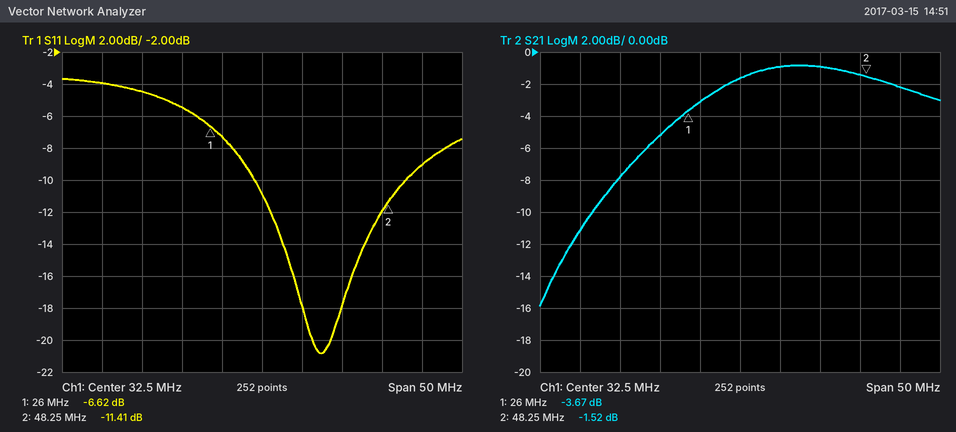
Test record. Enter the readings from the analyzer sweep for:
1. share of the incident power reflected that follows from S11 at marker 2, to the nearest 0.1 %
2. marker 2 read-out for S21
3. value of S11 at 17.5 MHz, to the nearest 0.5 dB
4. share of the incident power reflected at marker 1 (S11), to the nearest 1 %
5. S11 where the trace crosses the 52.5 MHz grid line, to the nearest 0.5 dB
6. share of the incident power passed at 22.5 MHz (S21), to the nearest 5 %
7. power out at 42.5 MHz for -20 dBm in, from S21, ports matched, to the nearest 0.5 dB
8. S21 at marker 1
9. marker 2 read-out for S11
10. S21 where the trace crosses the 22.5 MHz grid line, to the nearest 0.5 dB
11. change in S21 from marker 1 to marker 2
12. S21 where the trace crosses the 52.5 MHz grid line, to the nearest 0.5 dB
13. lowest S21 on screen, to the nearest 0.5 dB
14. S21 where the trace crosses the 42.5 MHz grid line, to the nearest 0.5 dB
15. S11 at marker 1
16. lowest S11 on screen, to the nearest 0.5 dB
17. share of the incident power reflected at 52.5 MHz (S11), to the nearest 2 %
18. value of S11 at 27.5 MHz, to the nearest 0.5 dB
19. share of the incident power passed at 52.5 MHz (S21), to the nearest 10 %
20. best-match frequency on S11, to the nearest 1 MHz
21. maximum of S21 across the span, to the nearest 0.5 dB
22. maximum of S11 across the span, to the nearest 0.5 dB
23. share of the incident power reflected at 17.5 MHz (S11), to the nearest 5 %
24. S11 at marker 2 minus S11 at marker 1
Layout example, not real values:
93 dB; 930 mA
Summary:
7.2 %; -1.52 dB; -4.5 dB; 22 %; -9.0 dB; 30 %; -21.0 dBm; -3.67 dB; -11.41 dB; -5.0 dB; 2.15 dB; -2.0 dB; -16.0 dB; -1.0 dB; -6.62 dB; -21.0 dB; 12 %; -7.5 dB; 60 %; 40 MHz; -1.0 dB; -3.5 dB; 35 %; -4.79 dB
